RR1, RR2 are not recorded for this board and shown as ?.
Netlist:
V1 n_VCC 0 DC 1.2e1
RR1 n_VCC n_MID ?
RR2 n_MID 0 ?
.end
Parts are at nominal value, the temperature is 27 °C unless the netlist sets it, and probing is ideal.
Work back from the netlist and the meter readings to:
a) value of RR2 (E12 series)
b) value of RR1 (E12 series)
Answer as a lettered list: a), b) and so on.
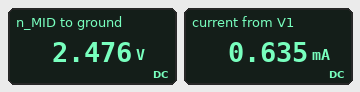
a) 3.9 kΩ
b) 15 kΩ
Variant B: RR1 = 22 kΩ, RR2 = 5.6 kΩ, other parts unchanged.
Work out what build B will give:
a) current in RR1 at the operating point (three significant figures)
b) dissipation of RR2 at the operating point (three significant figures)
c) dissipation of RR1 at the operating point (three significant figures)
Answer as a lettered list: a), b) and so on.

a) 435 µA
b) 1.06 mW
c) 4.16 mW
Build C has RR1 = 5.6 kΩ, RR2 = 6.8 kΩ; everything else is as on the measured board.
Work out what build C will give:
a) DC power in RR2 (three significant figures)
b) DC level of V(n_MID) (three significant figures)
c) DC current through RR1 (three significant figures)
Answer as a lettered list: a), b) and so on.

a) 6.37 mW
b) 6.58 V
c) 968 µA
